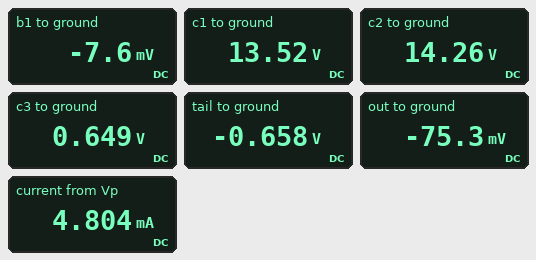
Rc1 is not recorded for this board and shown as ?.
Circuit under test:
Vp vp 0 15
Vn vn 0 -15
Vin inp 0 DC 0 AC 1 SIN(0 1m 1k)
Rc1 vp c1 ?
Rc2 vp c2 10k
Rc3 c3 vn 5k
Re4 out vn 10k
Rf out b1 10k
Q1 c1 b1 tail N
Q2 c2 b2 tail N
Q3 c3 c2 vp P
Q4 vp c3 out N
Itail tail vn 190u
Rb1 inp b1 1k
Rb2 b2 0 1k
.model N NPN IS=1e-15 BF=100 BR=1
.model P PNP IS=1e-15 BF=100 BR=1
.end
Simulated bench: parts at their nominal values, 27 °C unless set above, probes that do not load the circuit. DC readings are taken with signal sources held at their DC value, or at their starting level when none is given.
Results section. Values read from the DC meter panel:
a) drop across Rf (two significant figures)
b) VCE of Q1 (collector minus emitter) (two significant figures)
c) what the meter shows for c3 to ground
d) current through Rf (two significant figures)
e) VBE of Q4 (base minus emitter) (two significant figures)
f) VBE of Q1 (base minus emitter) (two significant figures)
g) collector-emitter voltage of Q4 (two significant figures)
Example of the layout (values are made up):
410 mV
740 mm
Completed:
68 mV
14 V
0.649 V
6.8 µA
720 mV
650 mV
15 V
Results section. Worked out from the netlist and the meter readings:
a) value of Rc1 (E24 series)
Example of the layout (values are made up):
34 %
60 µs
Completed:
18 kΩ
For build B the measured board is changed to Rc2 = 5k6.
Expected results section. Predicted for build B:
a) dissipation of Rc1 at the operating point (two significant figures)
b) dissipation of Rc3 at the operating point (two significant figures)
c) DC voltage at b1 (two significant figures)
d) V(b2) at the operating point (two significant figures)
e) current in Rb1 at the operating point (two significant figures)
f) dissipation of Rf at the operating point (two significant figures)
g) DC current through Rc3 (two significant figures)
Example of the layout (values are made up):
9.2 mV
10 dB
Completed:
11 µW
46 mW
-50 mV
-1.6 mV
50 µA
25 µW
3.0 mA
